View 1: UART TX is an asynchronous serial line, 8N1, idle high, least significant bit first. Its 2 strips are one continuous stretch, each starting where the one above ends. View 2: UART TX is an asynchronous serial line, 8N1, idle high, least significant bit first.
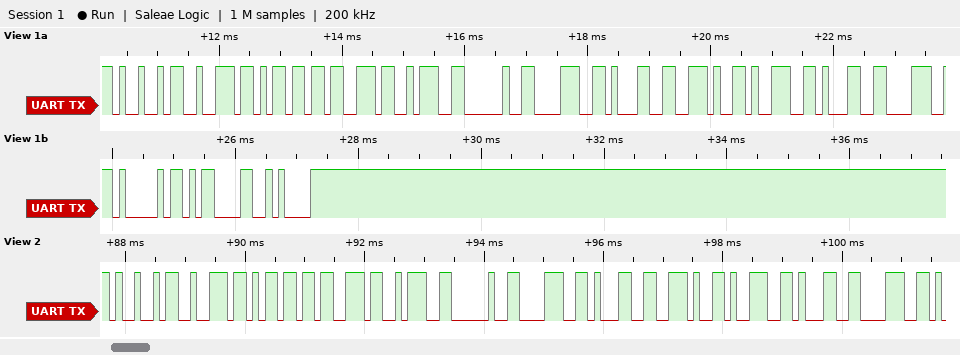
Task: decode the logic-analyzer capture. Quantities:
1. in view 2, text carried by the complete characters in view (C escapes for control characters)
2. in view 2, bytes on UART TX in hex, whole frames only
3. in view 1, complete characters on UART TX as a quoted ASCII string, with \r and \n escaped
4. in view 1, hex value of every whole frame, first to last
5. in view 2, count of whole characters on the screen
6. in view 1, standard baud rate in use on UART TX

"Irms: 81.918"
0x49 0x72 0x6D 0x73 0x3A 0x20 0x38 0x31 0x2E 0x39 0x31 0x38
"Irms: 81.918A\r\n"
49 72 6D 73 3A 20 38 31 2E 39 31 38 41 0D 0A
12
9600 baud
